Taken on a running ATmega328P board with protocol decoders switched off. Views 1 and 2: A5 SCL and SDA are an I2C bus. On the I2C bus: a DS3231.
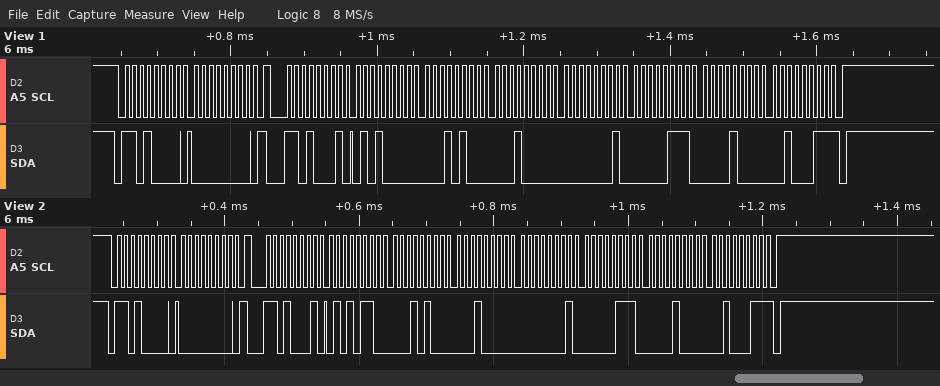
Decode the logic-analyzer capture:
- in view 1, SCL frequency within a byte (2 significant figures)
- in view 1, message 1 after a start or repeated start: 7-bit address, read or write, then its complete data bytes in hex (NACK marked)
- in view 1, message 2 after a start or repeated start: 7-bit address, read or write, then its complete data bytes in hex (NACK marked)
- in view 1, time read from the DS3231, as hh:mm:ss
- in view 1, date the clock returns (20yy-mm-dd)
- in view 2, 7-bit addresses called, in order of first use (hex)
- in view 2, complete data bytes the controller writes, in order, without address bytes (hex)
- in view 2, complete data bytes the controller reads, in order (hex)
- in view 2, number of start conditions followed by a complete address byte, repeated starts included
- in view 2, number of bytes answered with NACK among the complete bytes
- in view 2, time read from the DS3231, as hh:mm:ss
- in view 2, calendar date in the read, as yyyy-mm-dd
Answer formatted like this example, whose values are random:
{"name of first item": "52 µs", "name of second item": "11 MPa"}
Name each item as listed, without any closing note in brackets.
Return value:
{"in view 1, SCL frequency within a byte": "100 kHz", "in view 1, message 1 after a start or repeated start: 7-bit address, read or write, then its complete data bytes in hex": "0x68 write: 00", "in view 1, message 2 after a start or repeated start: 7-bit address, read or write, then its complete data bytes in hex": "0x68 read: 50 14 10 01 07 08 23 NACK", "in view 1, time read from the DS3231, as hh:mm:ss": "10:14:50", "in view 1, date the clock returns": "2023-08-07", "in view 2, 7-bit addresses called, in order of first use": "0x68", "in view 2, complete data bytes the controller writes, in order, without address bytes": "00", "in view 2, complete data bytes the controller reads, in order": "56 14 10 01 07 08 23", "in view 2, number of start conditions followed by a complete address byte, repeated starts included": "2", "in view 2, number of bytes answered with NACK among the complete bytes": "1", "in view 2, time read from the DS3231, as hh:mm:ss": "10:14:56", "in view 2, calendar date in the read, as yyyy-mm-dd": "2023-08-07"}
